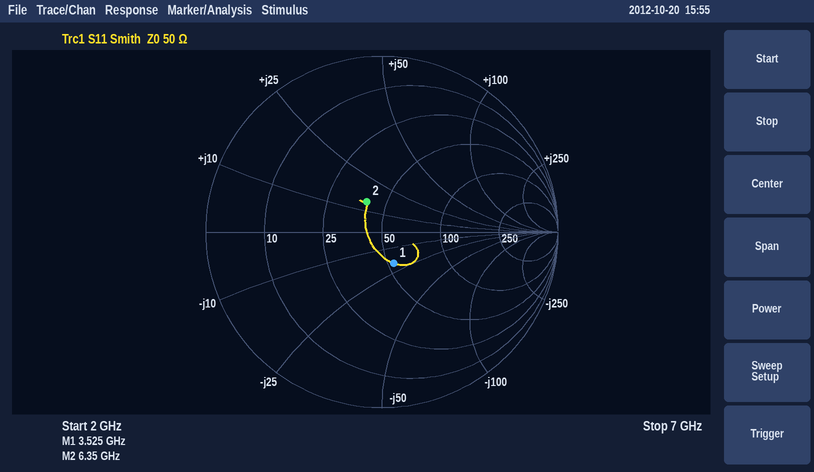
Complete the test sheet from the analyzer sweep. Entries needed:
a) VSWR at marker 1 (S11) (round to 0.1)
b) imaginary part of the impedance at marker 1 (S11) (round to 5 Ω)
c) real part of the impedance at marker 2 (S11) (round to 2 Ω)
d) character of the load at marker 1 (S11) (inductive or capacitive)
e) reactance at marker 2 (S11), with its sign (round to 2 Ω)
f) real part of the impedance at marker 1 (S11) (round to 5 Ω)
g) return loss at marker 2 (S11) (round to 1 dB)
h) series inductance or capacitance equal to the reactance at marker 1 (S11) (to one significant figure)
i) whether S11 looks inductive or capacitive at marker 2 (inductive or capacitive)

1.5
-20 Ω
40 Ω
capacitive
+14 Ω
55 Ω
14 dB
2 pF
inductive
